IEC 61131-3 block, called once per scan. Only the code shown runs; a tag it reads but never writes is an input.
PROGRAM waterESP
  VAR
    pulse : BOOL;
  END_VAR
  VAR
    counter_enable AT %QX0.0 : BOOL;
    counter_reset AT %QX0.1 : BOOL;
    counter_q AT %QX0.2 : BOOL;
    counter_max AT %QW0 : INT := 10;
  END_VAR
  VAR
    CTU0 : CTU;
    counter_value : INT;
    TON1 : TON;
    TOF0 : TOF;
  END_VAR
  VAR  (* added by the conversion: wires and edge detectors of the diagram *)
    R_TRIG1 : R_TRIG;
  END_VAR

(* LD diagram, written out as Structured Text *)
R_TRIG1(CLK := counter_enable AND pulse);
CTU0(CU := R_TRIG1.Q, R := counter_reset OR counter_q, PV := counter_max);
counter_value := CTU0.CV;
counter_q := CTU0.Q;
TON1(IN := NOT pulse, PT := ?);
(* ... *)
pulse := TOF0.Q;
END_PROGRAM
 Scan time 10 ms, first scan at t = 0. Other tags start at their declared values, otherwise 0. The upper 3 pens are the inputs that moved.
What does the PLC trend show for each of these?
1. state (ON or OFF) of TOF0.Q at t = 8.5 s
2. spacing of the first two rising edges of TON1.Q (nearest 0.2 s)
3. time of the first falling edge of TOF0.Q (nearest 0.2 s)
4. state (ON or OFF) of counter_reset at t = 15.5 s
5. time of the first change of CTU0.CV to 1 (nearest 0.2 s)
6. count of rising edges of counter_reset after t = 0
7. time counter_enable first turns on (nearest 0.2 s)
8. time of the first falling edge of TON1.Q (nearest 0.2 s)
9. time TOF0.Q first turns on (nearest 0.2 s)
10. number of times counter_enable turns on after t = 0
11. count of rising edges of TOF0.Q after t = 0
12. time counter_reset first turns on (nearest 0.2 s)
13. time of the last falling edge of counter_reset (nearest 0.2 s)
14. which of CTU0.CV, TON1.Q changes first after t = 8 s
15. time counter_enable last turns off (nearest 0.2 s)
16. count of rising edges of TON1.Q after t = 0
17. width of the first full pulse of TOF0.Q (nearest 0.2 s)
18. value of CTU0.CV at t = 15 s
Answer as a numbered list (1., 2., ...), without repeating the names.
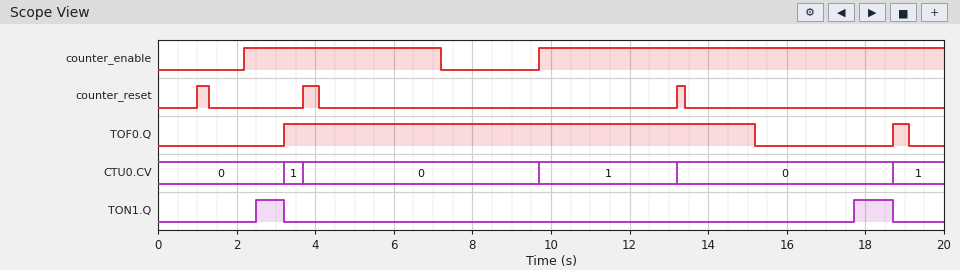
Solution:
1. ON
2. 15.2 s
3. 15.2 s
4. OFF
5. 3.2 s
6. 3
7. 2.2 s
8. 3.2 s
9. 3.2 s
10. 2
11. 2
12. 1.0 s
13. 13.4 s
14. CTU0.CV
15. 7.2 s
16. 2
17. 12.0 s
18. 0
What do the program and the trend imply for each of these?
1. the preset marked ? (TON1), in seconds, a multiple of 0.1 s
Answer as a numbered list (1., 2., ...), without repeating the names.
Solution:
1. 2.5 s
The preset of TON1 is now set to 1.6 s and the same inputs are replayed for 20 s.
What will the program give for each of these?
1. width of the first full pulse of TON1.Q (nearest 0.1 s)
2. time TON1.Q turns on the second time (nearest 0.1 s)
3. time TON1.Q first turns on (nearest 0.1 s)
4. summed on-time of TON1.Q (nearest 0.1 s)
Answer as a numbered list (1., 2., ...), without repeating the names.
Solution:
1. 1.6 s
2. 16.8 s
3. 1.6 s
4. 3.5 s
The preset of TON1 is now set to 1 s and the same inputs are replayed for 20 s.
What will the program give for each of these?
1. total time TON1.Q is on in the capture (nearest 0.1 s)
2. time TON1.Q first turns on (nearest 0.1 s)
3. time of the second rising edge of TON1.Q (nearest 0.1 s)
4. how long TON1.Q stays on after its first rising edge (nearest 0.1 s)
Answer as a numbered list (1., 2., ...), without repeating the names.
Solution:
1. 4.7 s
2. 1.0 s
3. 16.2 s
4. 2.2 s
